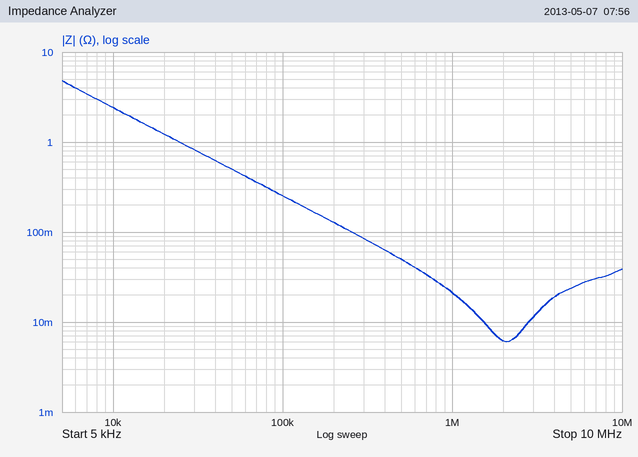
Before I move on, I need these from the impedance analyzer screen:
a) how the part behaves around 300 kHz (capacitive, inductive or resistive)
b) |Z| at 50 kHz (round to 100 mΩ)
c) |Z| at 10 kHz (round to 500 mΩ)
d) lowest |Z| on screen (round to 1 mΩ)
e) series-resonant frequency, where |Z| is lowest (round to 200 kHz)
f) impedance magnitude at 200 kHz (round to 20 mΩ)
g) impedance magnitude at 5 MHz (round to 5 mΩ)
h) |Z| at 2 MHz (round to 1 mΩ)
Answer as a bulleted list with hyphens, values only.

- capacitive
- 500 mΩ
- 2.5 Ω
- 6 mΩ
- 2.0 MHz
- 120 mΩ
- 25 mΩ
- 6 mΩ
